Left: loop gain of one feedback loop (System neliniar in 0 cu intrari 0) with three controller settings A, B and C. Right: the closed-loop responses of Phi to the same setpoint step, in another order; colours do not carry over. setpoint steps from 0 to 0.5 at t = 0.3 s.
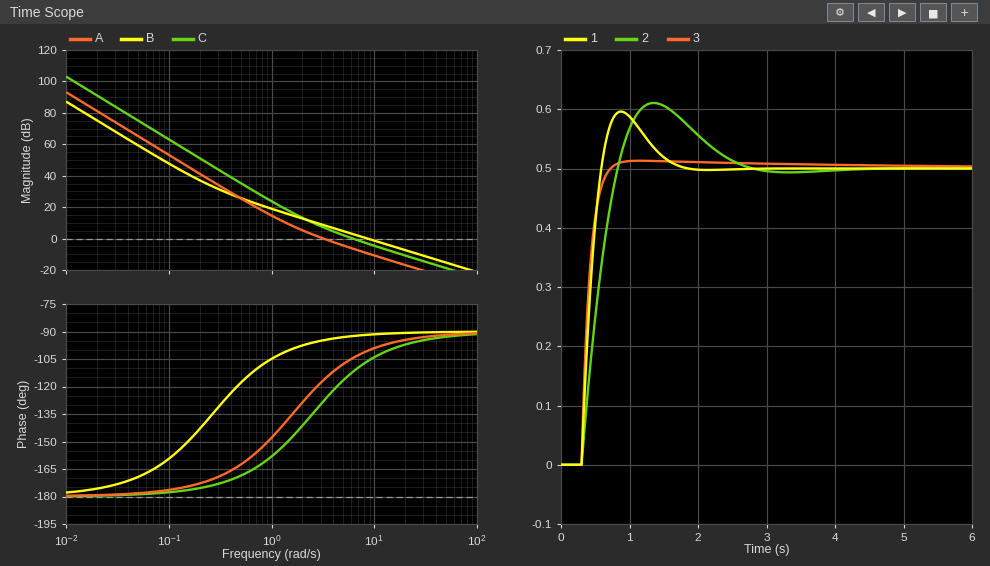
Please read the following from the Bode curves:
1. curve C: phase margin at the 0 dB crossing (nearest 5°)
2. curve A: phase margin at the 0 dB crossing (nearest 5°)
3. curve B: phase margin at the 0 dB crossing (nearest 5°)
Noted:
70°
65°
90°
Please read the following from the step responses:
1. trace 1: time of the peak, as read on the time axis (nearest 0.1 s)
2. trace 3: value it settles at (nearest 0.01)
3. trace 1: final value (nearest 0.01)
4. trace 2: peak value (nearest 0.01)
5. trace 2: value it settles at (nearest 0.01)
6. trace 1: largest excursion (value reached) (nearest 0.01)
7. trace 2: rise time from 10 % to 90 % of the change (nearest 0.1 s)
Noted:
0.9 s
0.50
0.50
0.61
0.50
0.60
0.4 s
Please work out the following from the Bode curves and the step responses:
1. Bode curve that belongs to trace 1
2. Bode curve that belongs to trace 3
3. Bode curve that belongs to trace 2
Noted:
C
B
A
